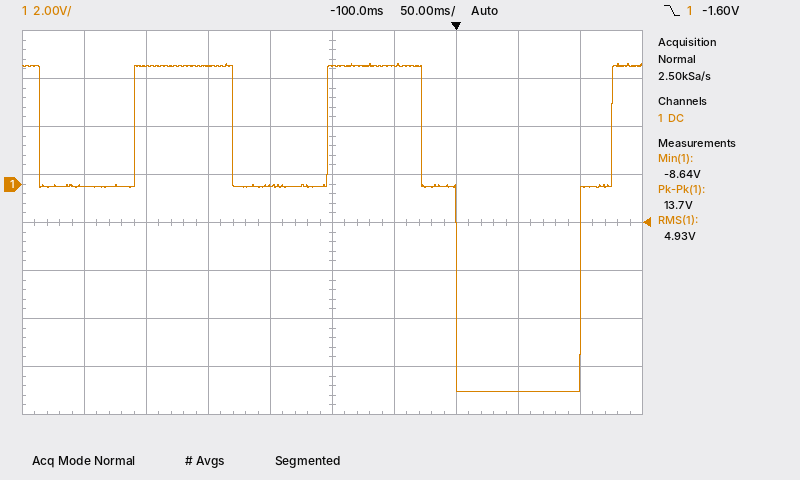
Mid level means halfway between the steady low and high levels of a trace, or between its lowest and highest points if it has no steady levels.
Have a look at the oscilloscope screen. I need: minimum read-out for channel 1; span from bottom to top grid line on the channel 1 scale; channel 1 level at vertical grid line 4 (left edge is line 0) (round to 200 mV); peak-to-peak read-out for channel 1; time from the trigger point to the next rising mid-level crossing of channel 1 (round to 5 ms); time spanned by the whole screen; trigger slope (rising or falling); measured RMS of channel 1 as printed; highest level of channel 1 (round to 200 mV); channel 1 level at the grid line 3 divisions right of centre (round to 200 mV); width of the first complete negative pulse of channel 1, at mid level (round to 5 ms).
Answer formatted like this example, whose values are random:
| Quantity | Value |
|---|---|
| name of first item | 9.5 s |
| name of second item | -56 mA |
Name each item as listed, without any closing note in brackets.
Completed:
| Quantity | Value |
|---|---|
| minimum read-out for channel 1 | -8.64 V |
| span from bottom to top grid line on the channel 1 scale | 16 V |
| channel 1 level at vertical grid line 4 (left edge is line 0) | 0.0 V |
| peak-to-peak read-out for channel 1 | 13.7 V |
| time from the trigger point to the next rising mid-level crossing of channel 1 | 100 ms |
| time spanned by the whole screen | 500 ms |
| trigger slope | falling |
| measured RMS of channel 1 as printed | 4.93 V |
| highest level of channel 1 | 5.0 V |
| channel 1 level at the grid line 3 divisions right of centre | -8.6 V |
| width of the first complete negative pulse of channel 1, at mid level | 100 ms |
